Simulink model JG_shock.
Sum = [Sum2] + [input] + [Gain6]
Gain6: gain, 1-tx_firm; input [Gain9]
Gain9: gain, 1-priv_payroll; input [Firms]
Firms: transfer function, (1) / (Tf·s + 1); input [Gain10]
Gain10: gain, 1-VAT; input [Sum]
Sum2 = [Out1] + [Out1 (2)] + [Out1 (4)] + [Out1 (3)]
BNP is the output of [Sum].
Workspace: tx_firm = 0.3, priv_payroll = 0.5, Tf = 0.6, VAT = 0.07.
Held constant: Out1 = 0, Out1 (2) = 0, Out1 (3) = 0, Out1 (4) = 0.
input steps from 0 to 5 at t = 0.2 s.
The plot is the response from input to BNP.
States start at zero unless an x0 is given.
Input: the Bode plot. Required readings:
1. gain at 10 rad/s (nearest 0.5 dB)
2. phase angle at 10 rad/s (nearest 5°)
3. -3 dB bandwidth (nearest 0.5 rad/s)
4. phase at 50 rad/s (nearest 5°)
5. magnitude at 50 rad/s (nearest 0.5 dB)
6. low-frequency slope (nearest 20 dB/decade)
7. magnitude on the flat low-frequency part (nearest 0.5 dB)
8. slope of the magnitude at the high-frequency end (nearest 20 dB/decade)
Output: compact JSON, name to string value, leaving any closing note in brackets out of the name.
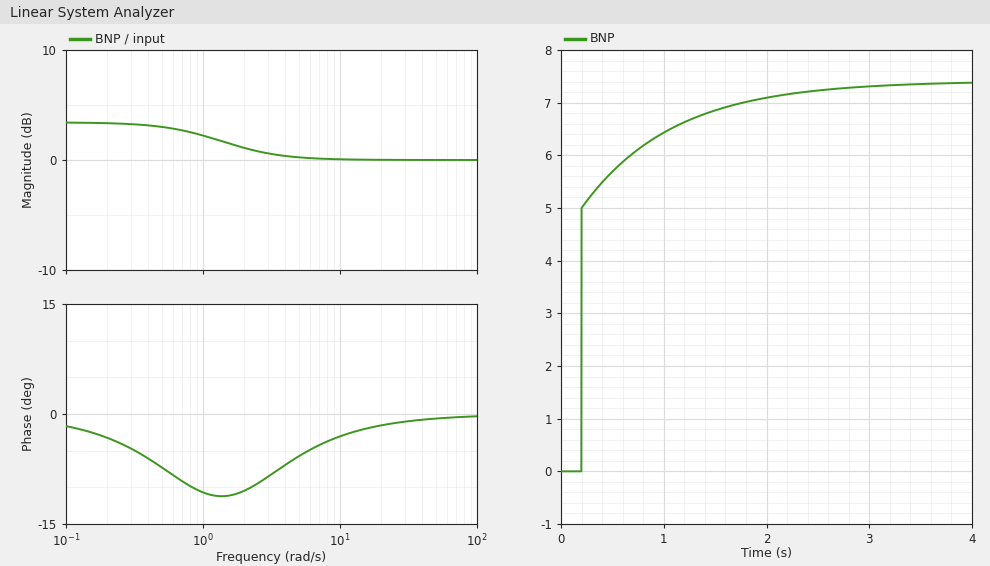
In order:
{"gain at 10 rad/s": "0.0 dB", "phase angle at 10 rad/s": "-5°", "-3 dB bandwidth": "4.0 rad/s", "phase at 50 rad/s": "0°", "magnitude at 50 rad/s": "0.0 dB", "low-frequency slope": "0 dB/decade", "magnitude on the flat low-frequency part": "3.5 dB", "slope of the magnitude at the high-frequency end": "0 dB/decade"}
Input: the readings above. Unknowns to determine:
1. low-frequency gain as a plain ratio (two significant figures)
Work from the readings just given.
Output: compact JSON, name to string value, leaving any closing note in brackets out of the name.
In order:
{"low-frequency gain as a plain ratio": "1.5"}
